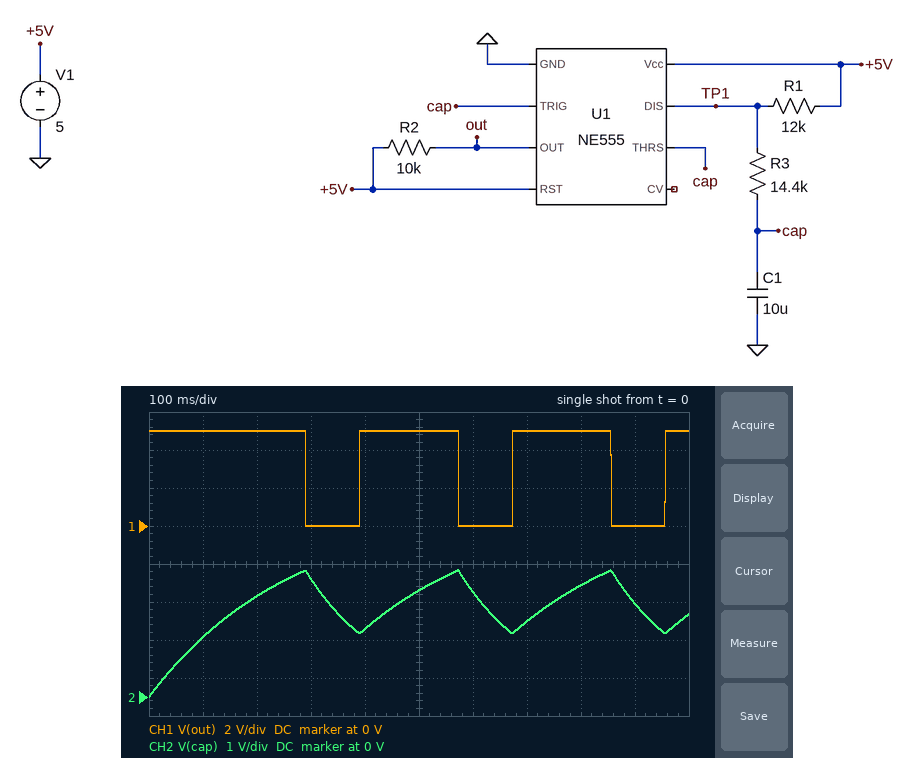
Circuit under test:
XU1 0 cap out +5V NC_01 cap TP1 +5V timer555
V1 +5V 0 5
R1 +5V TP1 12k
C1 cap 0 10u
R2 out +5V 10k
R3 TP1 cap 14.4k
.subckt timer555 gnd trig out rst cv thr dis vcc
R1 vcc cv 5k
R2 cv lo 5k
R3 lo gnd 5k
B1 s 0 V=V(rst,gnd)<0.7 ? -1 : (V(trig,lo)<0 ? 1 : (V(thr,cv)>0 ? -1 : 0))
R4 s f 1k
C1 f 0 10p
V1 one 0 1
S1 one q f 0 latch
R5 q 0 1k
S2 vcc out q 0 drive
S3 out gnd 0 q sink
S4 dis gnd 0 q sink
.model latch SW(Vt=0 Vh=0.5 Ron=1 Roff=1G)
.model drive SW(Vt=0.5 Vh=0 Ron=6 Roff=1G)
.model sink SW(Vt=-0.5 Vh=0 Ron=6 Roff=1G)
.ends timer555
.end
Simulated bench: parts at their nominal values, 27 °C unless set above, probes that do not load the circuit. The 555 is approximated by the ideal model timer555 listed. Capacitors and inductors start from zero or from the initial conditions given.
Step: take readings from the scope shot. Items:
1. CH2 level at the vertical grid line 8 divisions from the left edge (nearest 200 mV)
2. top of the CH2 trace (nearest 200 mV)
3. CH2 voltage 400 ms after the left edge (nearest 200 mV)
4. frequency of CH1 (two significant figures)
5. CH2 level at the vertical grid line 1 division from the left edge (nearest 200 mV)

3.0 V
3.4 V
1.8 V
3.5 Hz
1.6 V
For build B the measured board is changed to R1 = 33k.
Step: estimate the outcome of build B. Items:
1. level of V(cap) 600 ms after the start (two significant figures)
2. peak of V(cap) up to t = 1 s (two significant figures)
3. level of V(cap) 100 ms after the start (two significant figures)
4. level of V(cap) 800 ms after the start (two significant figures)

1.9 V
3.3 V
950 mV
2.7 V
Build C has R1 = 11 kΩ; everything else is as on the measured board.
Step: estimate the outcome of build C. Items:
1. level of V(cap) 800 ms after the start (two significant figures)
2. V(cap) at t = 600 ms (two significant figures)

3.1 V
2.4 V
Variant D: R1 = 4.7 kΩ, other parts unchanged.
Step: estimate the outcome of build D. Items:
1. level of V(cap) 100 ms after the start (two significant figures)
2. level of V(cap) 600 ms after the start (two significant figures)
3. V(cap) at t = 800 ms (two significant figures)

2.0 V
2.5 V
2.1 V
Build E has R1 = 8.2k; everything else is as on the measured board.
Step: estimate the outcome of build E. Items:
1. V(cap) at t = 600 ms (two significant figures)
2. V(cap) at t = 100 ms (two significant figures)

1.7 V
1.8 V
